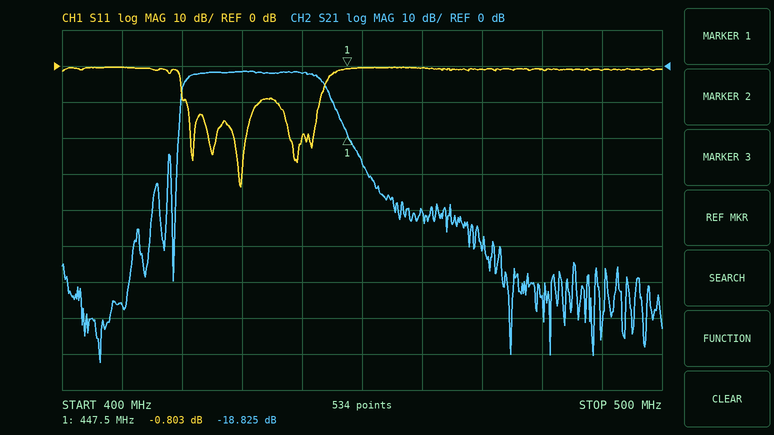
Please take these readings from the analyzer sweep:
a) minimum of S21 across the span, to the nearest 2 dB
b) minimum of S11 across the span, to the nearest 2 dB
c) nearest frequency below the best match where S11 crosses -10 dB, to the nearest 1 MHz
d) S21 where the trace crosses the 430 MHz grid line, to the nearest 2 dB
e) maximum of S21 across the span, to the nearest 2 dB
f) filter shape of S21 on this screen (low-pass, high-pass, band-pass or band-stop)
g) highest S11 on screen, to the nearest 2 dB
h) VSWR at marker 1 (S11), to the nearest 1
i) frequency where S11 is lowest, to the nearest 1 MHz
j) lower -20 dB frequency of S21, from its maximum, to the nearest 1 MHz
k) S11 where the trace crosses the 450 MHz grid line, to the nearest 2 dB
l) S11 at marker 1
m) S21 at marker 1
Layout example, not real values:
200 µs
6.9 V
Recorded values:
-82 dB
-34 dB
421 MHz
-2 dB
-2 dB
band-pass
0 dB
22
430 MHz
419 MHz
0 dB
-0.803 dB
-18.825 dB
